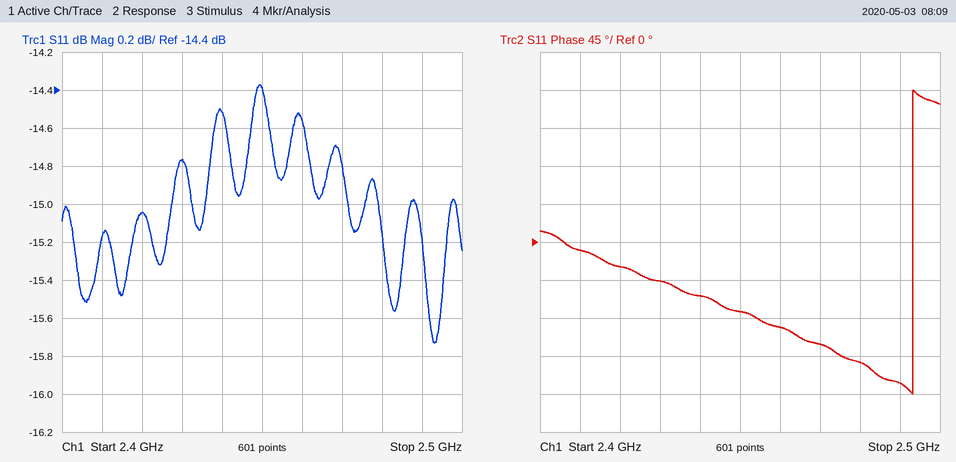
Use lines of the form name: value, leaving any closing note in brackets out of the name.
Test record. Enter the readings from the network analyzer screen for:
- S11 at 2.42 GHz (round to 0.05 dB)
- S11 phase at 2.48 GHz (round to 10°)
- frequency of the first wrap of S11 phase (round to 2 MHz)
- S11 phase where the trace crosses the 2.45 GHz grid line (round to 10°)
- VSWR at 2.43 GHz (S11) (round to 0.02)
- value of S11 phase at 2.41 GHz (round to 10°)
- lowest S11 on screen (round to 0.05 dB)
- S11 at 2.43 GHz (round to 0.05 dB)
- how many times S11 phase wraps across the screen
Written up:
S11 at 2.42 GHz: -15.05 dB
S11 phase at 2.48 GHz: -140°
frequency of the first wrap of S11 phase: 2.494 GHz
S11 phase where the trace crosses the 2.45 GHz grid line: -80°
VSWR at 2.43 GHz (S11): 1.44
value of S11 phase at 2.41 GHz: -10°
lowest S11 on screen: -15.75 dB
S11 at 2.43 GHz: -14.75 dB
how many times S11 phase wraps across the screen: 1
